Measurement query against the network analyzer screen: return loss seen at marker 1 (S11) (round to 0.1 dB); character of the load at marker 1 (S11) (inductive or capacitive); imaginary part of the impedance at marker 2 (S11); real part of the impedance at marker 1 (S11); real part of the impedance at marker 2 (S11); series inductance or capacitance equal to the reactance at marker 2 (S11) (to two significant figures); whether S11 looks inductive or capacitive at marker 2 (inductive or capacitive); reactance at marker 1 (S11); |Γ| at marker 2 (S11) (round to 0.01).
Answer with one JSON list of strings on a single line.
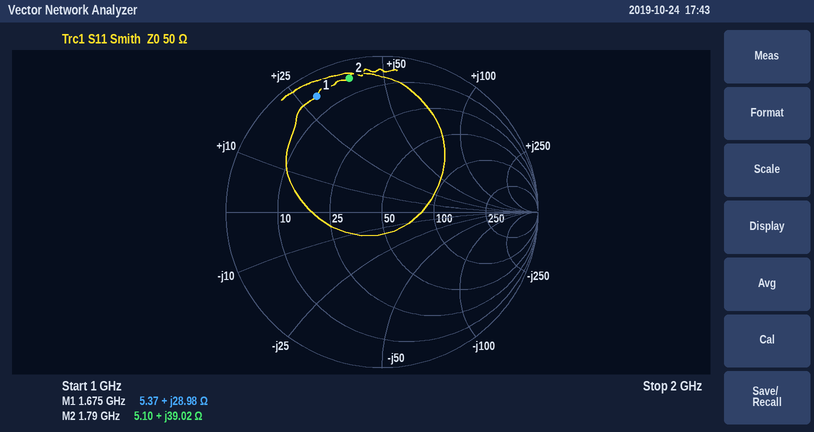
["1.4 dB", "inductive", "+39.02 Ω", "5.37 Ω", "5.10 Ω", "3.5 nH", "inductive", "+28.98 Ω", "0.88"]
